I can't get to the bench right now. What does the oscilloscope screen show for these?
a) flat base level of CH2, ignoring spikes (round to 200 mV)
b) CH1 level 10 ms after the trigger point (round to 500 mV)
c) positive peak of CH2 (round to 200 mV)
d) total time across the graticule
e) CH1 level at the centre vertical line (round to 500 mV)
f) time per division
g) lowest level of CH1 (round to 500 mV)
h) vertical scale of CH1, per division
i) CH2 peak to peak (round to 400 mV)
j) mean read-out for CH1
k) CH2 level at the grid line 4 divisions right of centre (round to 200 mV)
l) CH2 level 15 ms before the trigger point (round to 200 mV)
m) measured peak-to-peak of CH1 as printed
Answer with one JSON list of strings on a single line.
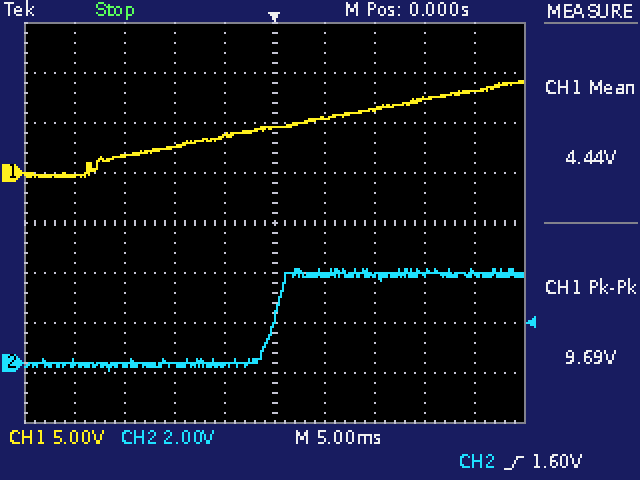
["0.0 V", "6.5 V", "3.8 V", "50 ms", "4.5 V", "5 ms", "-500 mV", "5 V", "4.0 V", "4.44 V", "3.6 V", "0.0 V", "9.69 V"]
